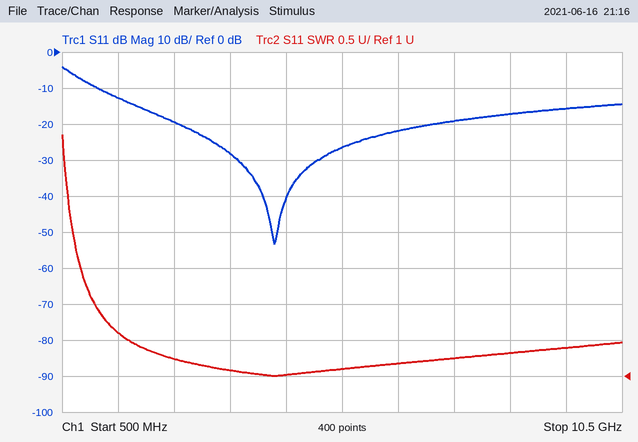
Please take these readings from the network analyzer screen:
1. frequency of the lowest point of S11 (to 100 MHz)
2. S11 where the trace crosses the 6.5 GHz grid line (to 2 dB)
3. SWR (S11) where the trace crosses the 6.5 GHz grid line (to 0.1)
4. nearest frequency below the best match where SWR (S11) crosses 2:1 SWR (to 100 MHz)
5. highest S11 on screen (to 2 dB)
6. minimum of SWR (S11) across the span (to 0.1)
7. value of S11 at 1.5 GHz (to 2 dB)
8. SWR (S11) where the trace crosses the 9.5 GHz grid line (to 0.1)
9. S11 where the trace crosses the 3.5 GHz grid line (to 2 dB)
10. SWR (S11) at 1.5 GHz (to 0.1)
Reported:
4.3 GHz
-22 dB
1.2
1.1 GHz
-4 dB
1.0
-12 dB
1.4
-28 dB
1.6
